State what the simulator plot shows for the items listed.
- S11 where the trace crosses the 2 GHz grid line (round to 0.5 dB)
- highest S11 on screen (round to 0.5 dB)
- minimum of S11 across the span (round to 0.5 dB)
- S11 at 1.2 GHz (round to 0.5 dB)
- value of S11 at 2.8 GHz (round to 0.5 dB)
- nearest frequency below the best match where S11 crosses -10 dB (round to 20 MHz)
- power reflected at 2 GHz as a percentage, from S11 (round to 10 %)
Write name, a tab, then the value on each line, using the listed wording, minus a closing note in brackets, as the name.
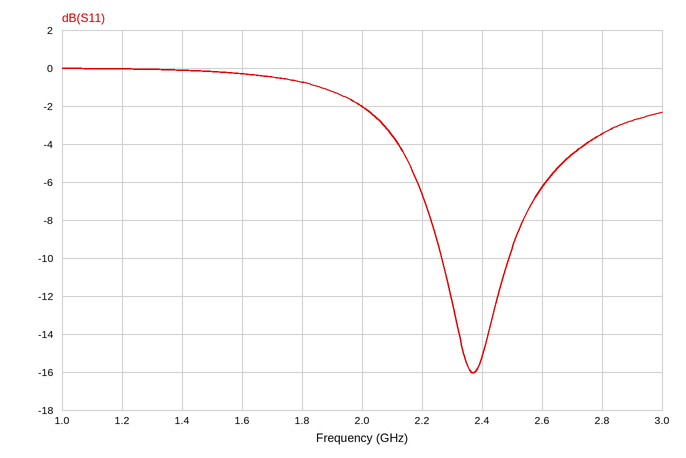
S11 where the trace crosses the 2 GHz grid line	-2.0 dB
highest S11 on screen	0.0 dB
minimum of S11 across the span	-16.0 dB
S11 at 1.2 GHz	0.0 dB
value of S11 at 2.8 GHz	-3.5 dB
nearest frequency below the best match where S11 crosses -10 dB	2.26 GHz
power reflected at 2 GHz as a percentage, from S11	60 %
